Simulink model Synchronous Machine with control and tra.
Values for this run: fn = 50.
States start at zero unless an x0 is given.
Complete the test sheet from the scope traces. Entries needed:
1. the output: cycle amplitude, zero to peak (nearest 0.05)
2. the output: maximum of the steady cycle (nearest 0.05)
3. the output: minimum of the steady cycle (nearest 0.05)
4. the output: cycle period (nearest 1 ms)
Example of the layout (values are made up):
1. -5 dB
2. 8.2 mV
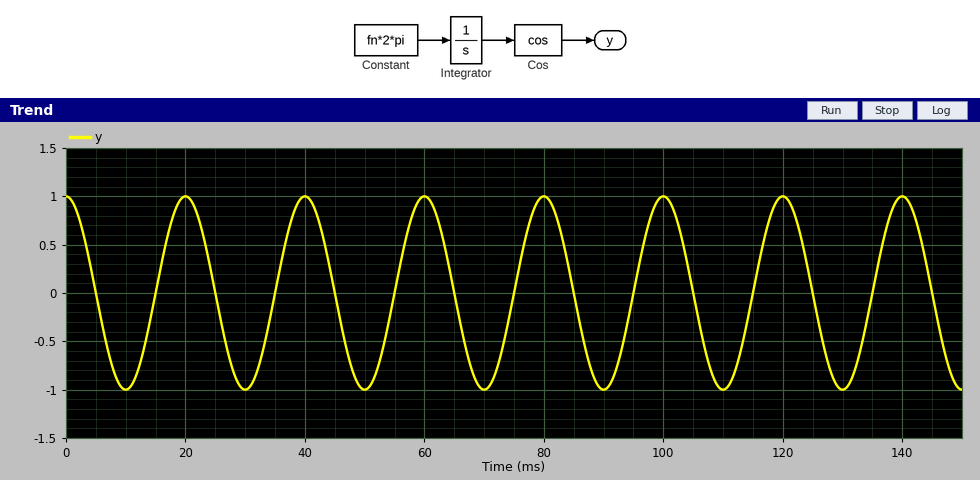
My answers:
1. 1.00
2. 1.00
3. -1.00
4. 20 ms
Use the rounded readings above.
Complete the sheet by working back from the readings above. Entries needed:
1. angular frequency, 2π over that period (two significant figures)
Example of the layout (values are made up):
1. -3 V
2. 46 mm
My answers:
1. 0.31 rad/ms
